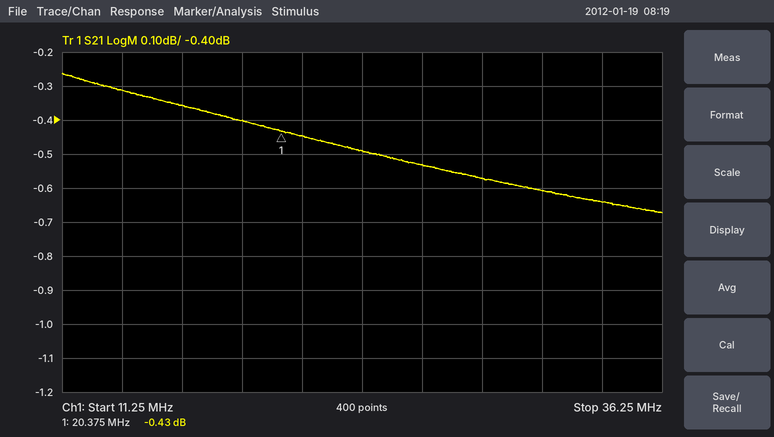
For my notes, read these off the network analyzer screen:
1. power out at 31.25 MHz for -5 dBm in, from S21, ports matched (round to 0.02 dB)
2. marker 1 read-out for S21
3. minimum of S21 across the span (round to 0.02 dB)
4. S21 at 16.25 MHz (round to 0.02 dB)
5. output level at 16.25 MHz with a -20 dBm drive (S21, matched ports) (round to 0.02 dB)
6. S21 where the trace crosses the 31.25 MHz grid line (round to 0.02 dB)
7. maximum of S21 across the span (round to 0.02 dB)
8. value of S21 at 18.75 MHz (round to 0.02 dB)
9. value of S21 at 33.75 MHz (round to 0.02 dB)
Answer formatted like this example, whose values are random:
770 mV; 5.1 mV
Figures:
-5.60 dBm; -0.43 dB; -0.68 dB; -0.36 dB; -20.36 dBm; -0.60 dB; -0.26 dB; -0.40 dB; -0.64 dB
